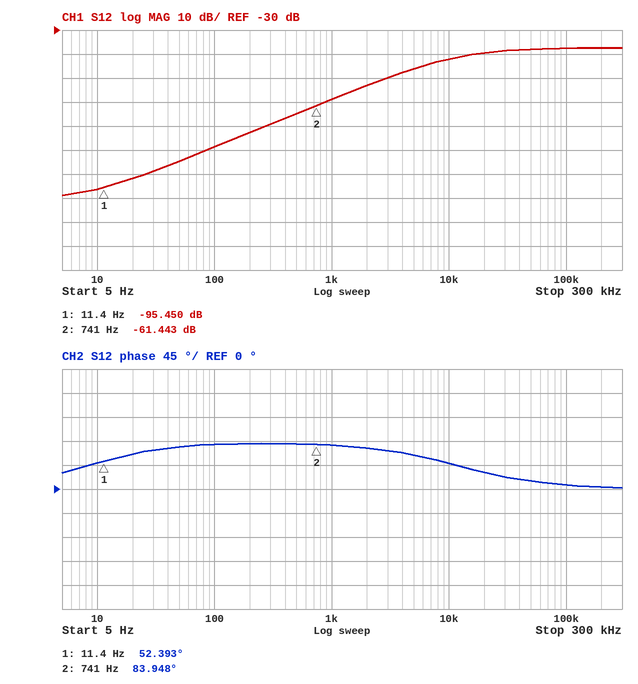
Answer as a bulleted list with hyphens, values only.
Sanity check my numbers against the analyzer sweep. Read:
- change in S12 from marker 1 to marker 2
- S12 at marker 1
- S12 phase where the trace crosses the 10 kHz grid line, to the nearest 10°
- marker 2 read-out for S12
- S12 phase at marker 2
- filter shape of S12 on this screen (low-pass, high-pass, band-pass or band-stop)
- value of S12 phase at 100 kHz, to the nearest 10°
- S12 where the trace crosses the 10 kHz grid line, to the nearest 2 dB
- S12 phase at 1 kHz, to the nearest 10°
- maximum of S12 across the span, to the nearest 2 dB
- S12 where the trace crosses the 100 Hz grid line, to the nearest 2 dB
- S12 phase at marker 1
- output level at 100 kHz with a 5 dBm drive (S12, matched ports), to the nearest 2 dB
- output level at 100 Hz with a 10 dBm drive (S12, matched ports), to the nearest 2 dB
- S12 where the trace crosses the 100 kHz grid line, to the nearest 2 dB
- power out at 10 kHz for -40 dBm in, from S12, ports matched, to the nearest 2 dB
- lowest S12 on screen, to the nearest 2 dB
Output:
- 34.007 dB
- -95.450 dB
- 50°
- -61.443 dB
- 83.948°
- high-pass
- 10°
- -42 dB
- 80°
- -38 dB
- -78 dB
- 52.393°
- -32 dBm
- -68 dBm
- -38 dB
- -82 dBm
- -98 dB
